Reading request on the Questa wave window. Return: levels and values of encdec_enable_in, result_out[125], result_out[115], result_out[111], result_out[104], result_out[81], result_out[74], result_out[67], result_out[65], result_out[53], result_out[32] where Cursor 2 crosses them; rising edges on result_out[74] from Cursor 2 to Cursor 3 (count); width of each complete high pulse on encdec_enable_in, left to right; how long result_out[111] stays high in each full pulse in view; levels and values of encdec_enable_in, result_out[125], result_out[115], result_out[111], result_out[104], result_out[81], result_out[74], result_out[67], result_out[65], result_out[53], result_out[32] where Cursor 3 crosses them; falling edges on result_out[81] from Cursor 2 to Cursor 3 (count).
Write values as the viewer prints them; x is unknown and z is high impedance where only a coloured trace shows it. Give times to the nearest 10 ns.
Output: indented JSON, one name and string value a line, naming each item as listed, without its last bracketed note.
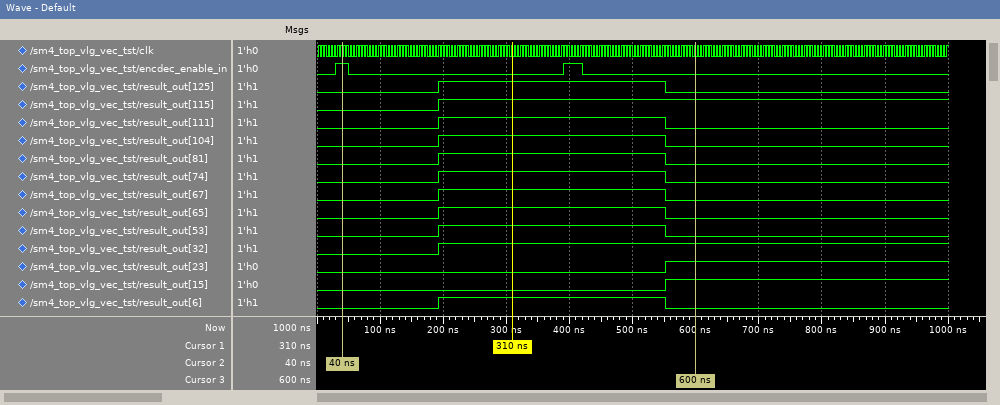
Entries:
{
  "levels and values of encdec_enable_in, result_out[125], result_out[115], result_out[111], result_out[104], result_out[81], result_out[74], result_out[67], result_out[65], result_out[53], result_out[32] where Cursor 2 crosses them": "encdec_enable_in=1, result_out[125]=0, result_out[115]=0, result_out[111]=0, result_out[104]=0, result_out[81]=0, result_out[74]=0, result_out[67]=0, result_out[65]=0, result_out[53]=0, result_out[32]=0",
  "rising edges on result_out[74] from Cursor 2 to Cursor 3": "1",
  "width of each complete high pulse on encdec_enable_in, left to right": "20 ns, 30 ns",
  "how long result_out[111] stays high in each full pulse in view": "360 ns",
  "levels and values of encdec_enable_in, result_out[125], result_out[115], result_out[111], result_out[104], result_out[81], result_out[74], result_out[67], result_out[65], result_out[53], result_out[32] where Cursor 3 crosses them": "encdec_enable_in=0, result_out[125]=0, result_out[115]=1, result_out[111]=0, result_out[104]=0, result_out[81]=0, result_out[74]=0, result_out[67]=0, result_out[65]=0, result_out[53]=0, result_out[32]=1",
  "falling edges on result_out[81] from Cursor 2 to Cursor 3": "1"
}
